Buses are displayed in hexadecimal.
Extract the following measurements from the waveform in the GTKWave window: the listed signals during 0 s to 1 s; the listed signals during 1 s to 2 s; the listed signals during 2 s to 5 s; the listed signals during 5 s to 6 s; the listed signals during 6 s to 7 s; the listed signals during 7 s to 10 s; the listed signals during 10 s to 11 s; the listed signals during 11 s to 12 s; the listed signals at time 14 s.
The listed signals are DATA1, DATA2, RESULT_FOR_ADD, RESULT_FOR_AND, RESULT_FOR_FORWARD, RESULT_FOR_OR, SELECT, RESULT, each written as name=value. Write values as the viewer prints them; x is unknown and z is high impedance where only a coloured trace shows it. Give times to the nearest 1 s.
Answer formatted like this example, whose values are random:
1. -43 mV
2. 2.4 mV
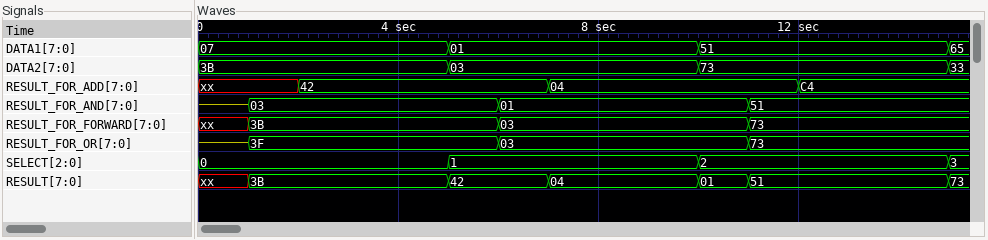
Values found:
1. DATA1=07, DATA2=3B, RESULT_FOR_ADD=xx, RESULT_FOR_AND=z, RESULT_FOR_FORWARD=xx, RESULT_FOR_OR=z, SELECT=0, RESULT=xx
2. DATA1=07, DATA2=3B, RESULT_FOR_ADD=xx, RESULT_FOR_AND=03, RESULT_FOR_FORWARD=3B, RESULT_FOR_OR=3F, SELECT=0, RESULT=3B
3. DATA1=07, DATA2=3B, RESULT_FOR_ADD=42, RESULT_FOR_AND=03, RESULT_FOR_FORWARD=3B, RESULT_FOR_OR=3F, SELECT=0, RESULT=3B
4. DATA1=01, DATA2=03, RESULT_FOR_ADD=42, RESULT_FOR_AND=03, RESULT_FOR_FORWARD=3B, RESULT_FOR_OR=3F, SELECT=1, RESULT=42
5. DATA1=01, DATA2=03, RESULT_FOR_ADD=42, RESULT_FOR_AND=01, RESULT_FOR_FORWARD=03, RESULT_FOR_OR=03, SELECT=1, RESULT=42
6. DATA1=01, DATA2=03, RESULT_FOR_ADD=04, RESULT_FOR_AND=01, RESULT_FOR_FORWARD=03, RESULT_FOR_OR=03, SELECT=1, RESULT=04
7. DATA1=51, DATA2=73, RESULT_FOR_ADD=04, RESULT_FOR_AND=01, RESULT_FOR_FORWARD=03, RESULT_FOR_OR=03, SELECT=2, RESULT=01
8. DATA1=51, DATA2=73, RESULT_FOR_ADD=04, RESULT_FOR_AND=51, RESULT_FOR_FORWARD=73, RESULT_FOR_OR=73, SELECT=2, RESULT=51
9. DATA1=51, DATA2=73, RESULT_FOR_ADD=C4, RESULT_FOR_AND=51, RESULT_FOR_FORWARD=73, RESULT_FOR_OR=73, SELECT=2, RESULT=51
